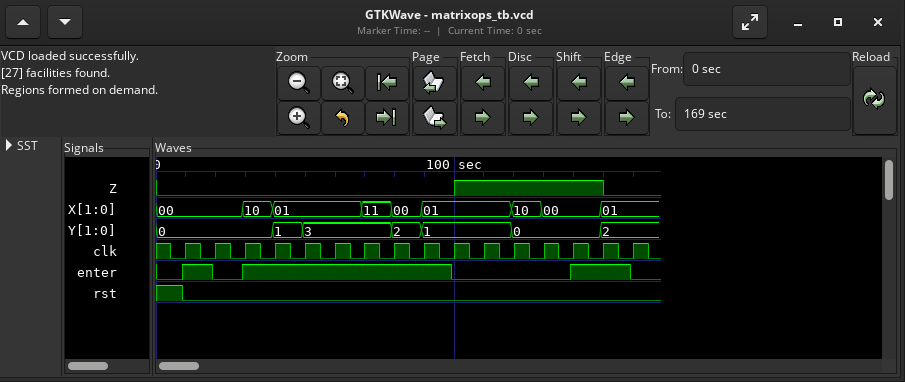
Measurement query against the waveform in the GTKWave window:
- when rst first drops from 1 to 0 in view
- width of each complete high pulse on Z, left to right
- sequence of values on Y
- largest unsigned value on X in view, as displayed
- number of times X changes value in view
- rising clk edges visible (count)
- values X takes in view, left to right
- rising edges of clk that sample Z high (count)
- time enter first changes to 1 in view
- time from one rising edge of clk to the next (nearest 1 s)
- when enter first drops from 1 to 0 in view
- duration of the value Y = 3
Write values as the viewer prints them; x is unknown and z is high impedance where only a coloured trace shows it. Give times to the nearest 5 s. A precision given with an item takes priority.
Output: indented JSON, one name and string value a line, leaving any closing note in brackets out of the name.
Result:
{
  "when rst first drops from 1 to 0 in view": "10 s",
  "width of each complete high pulse on Z, left to right": "50 s",
  "sequence of values on Y": "0, 1, 3, 2, 1, 0, 2",
  "largest unsigned value on X in view, as displayed": "11",
  "number of times X changes value in view": "8",
  "rising clk edges visible": "16",
  "values X takes in view, left to right": "00, 10, 01, 11, 00, 01, 10, 00, 01",
  "rising edges of clk that sample Z high": "5",
  "time enter first changes to 1 in view": "10 s",
  "time from one rising edge of clk to the next": "10 s",
  "when enter first drops from 1 to 0 in view": "20 s",
  "duration of the value Y = 3": "30 s"
}
